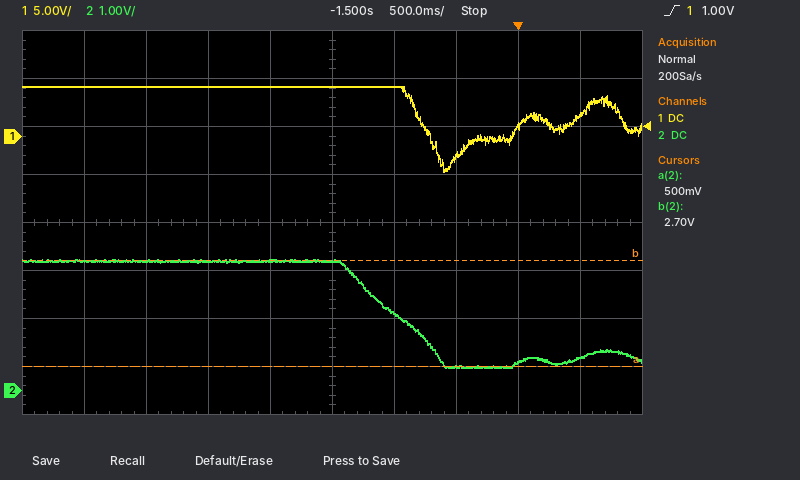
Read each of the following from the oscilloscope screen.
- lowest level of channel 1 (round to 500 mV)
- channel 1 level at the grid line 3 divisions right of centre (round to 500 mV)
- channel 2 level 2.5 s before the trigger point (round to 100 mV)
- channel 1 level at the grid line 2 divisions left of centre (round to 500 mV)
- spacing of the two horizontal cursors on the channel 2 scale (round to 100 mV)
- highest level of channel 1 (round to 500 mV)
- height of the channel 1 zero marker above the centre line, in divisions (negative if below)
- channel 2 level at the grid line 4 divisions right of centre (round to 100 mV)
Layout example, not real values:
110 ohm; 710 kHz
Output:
-3.5 V; 1.0 V; 2.7 V; 5.0 V; 2.2 V; 5.0 V; +1.8 div; 700 mV
